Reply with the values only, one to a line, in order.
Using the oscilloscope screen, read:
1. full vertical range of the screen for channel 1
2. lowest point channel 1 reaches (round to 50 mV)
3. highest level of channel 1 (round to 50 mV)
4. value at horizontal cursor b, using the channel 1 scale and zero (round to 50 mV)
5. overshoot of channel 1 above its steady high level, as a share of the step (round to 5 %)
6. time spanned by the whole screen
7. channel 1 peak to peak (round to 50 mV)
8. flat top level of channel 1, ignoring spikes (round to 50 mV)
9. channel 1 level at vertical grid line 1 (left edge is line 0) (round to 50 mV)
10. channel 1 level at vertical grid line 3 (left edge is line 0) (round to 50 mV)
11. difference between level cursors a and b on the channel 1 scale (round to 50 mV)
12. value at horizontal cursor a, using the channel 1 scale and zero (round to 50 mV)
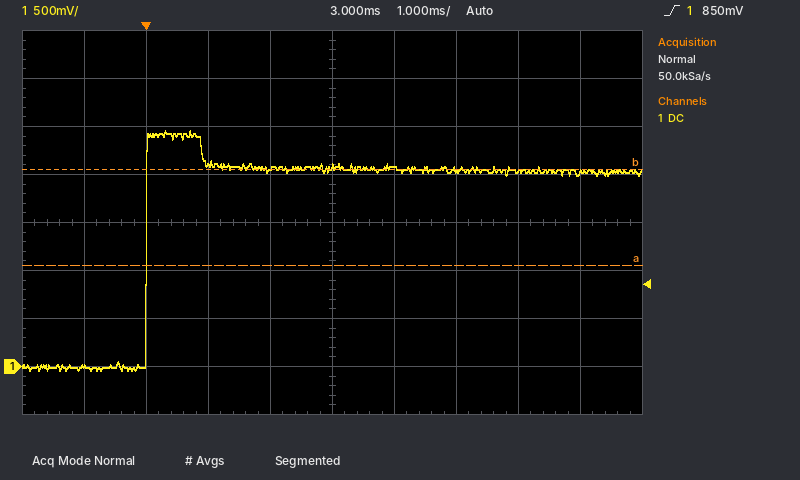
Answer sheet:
4 V
-50 mV
2.45 V
2.05 V
20 %
10 ms
2.50 V
2.05 V
0 mV
2.10 V
1.00 V
1.05 V
